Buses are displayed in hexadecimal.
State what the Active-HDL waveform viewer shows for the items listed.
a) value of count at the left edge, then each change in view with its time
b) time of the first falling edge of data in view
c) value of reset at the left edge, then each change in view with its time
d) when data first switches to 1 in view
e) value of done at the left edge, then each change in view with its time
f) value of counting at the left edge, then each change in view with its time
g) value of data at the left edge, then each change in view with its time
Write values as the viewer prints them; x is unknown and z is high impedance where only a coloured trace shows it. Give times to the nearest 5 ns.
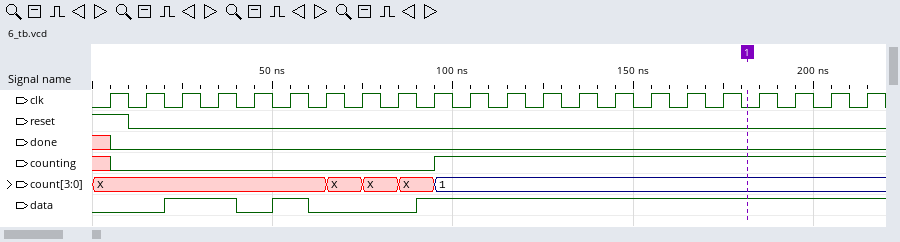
X, X at 65 ns, X at 75 ns, X at 85 ns, 1 at 95 ns
40 ns
1, 0 at 10 ns
20 ns
x, 0 at 5 ns
x, 0 at 5 ns, 1 at 95 ns
0, 1 at 20 ns, 0 at 40 ns, 1 at 50 ns, 0 at 60 ns, 1 at 90 ns
